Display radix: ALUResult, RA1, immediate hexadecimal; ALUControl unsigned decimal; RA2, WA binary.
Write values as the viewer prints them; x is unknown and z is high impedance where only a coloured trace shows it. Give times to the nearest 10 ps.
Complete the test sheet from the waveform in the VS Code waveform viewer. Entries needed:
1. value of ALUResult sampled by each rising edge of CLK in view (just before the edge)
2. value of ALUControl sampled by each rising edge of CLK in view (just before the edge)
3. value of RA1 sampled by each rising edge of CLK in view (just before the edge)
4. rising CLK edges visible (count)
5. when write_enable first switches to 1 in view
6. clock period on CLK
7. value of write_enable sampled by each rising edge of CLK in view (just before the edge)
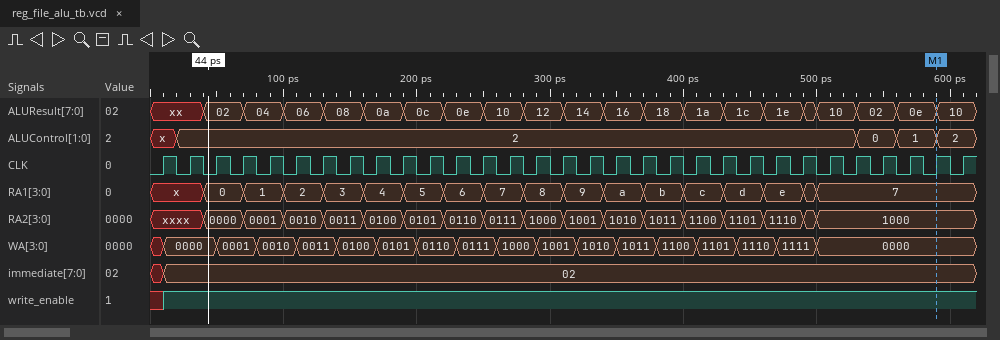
xx, xx, 02, 02, 04, 06, 06, 08, 0a, 0a, 0c, 0e, 0e, 10, 12, 12, 14, 16, 16, 18, 1a, 1a, 1c, 1e, 1e, 10, 10, 02, 0e, 0e, 10
x, 2, 2, 2, 2, 2, 2, 2, 2, 2, 2, 2, 2, 2, 2, 2, 2, 2, 2, 2, 2, 2, 2, 2, 2, 2, 2, 0, 1, 1, 2
x, x, 0, 0, 1, 2, 2, 3, 4, 4, 5, 6, 6, 7, 8, 8, 9, a, a, b, c, c, d, e, e, 7, 7, 7, 7, 7, 7
31
10 ps
20 ps
x 1 1 1 1 1 1 1 1 1 1 1 1 1 1 1 1 1 1 1 1 1 1 1 1 1 1 1 1 1 1
